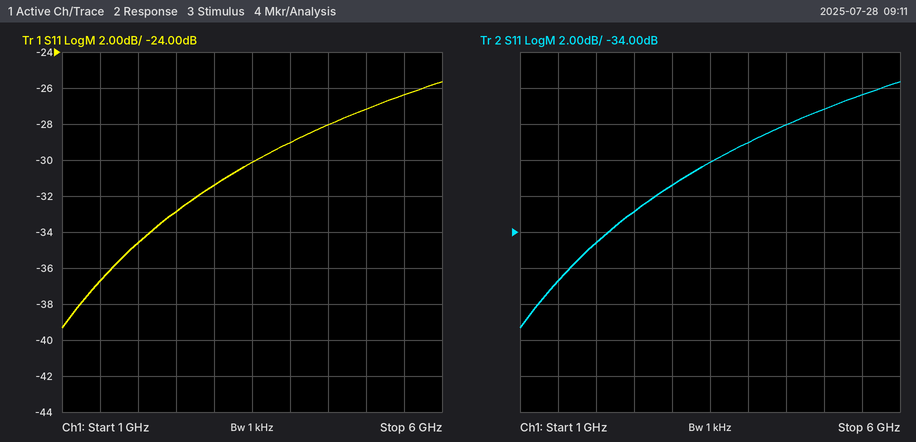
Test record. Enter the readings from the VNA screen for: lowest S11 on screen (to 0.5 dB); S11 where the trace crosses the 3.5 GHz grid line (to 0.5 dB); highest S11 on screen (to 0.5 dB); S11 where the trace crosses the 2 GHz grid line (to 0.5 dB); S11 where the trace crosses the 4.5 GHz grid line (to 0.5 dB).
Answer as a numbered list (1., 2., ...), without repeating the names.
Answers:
1. -39.5 dB
2. -30.0 dB
3. -25.5 dB
4. -34.5 dB
5. -28.0 dB
